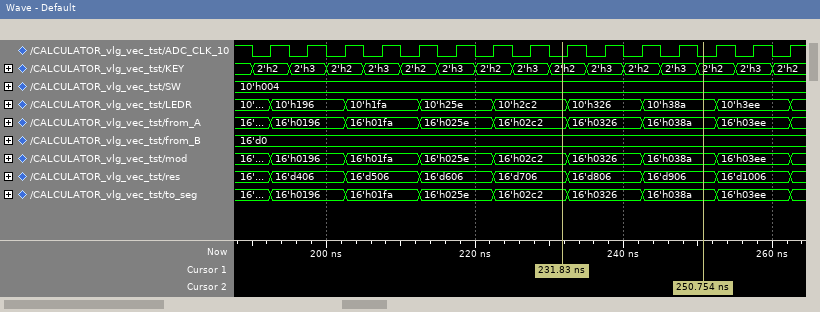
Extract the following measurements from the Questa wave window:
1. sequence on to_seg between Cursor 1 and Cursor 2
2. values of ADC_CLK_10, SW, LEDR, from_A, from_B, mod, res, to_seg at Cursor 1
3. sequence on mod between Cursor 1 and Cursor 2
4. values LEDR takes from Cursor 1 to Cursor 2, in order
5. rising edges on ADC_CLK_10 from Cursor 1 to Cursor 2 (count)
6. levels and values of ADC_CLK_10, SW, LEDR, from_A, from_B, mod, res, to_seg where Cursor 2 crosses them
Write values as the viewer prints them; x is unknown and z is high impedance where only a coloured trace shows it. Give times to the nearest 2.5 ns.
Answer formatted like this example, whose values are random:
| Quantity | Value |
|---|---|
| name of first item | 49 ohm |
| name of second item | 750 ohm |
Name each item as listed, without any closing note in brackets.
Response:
| Quantity | Value |
|---|---|
| sequence on to_seg between Cursor 1 and Cursor 2 | 16'h02c2, 16'h0326, 16'h038a |
| values of ADC_CLK_10, SW, LEDR, from_A, from_B, mod, res, to_seg at Cursor 1 | ADC_CLK_10=0, SW=10'h004, LEDR=10'h2c2, from_A=16'h02c2, from_B=16'd0, mod=16'h02c2, res=16'd706, to_seg=16'h02c2 |
| sequence on mod between Cursor 1 and Cursor 2 | 16'h02c2, 16'h0326, 16'h038a |
| values LEDR takes from Cursor 1 to Cursor 2, in order | 10'h2c2, 10'h326, 10'h38a |
| rising edges on ADC_CLK_10 from Cursor 1 to Cursor 2 | 4 |
| levels and values of ADC_CLK_10, SW, LEDR, from_A, from_B, mod, res, to_seg where Cursor 2 crosses them | ADC_CLK_10=0, SW=10'h004, LEDR=10'h38a, from_A=16'h038a, from_B=16'd0, mod=16'h038a, res=16'd906, to_seg=16'h038a |
